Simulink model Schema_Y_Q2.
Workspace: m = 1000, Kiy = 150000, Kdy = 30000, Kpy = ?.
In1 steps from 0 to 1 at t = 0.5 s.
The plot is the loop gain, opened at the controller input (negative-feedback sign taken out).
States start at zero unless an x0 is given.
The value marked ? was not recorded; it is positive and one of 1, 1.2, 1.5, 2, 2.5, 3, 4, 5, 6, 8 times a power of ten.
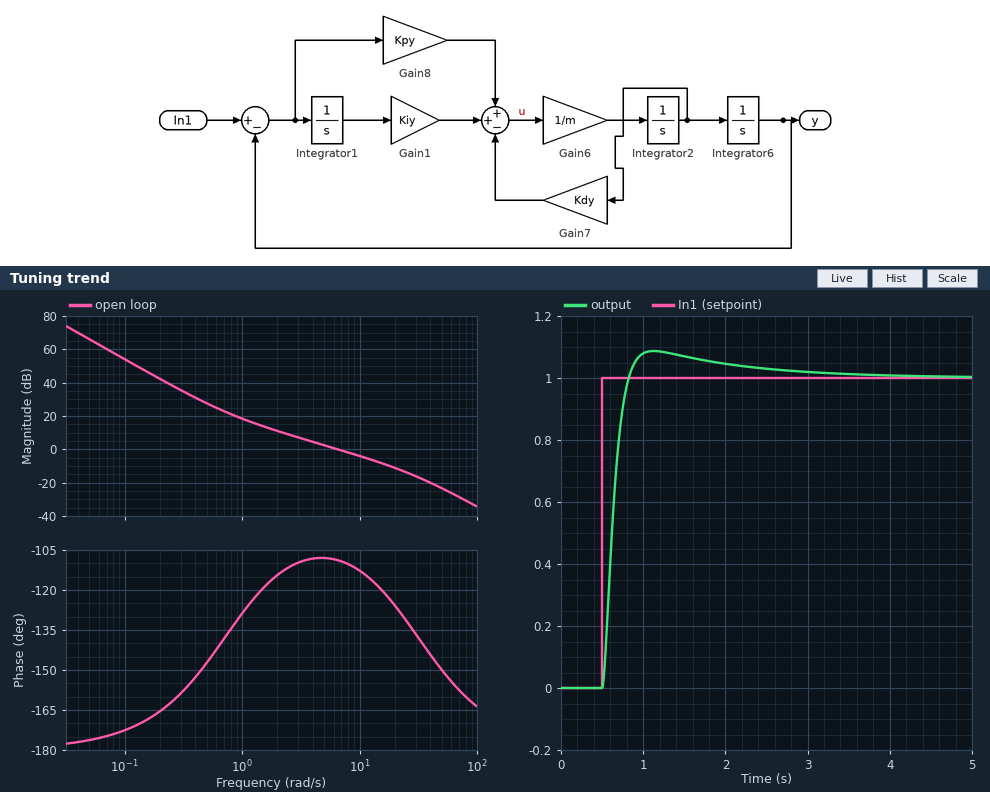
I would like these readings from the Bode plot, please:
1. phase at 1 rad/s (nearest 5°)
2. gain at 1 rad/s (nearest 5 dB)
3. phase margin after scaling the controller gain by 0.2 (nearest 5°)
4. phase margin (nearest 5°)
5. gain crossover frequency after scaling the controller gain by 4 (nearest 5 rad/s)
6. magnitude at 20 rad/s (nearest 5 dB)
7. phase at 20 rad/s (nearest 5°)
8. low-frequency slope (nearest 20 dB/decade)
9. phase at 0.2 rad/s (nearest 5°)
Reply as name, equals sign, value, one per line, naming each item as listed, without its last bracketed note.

phase at 1 rad/s = -130°
gain at 1 rad/s = 20 dB
phase margin after scaling the controller gain by 0.2 = 60°
phase margin = 70°
gain crossover frequency after scaling the controller gain by 4 = 20 rad/s
magnitude at 20 rad/s = -10 dB
phase at 20 rad/s = -125°
low-frequency slope = -40 dB/decade
phase at 0.2 rad/s = -165°
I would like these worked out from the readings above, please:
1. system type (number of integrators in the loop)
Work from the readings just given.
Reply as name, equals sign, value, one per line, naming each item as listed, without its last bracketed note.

system type = 2
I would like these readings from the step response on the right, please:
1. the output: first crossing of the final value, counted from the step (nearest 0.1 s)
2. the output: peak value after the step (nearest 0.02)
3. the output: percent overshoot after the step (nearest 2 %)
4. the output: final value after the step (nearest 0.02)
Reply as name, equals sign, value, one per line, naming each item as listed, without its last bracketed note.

the output: first crossing of the final value, counted from the step = 0.3 s
the output: peak value after the step = 1.08
the output: percent overshoot after the step = 8 %
the output: final value after the step = 1.00
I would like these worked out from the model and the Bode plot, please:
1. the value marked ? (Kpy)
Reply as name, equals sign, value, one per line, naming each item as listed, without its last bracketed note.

the value marked ? = 200000
